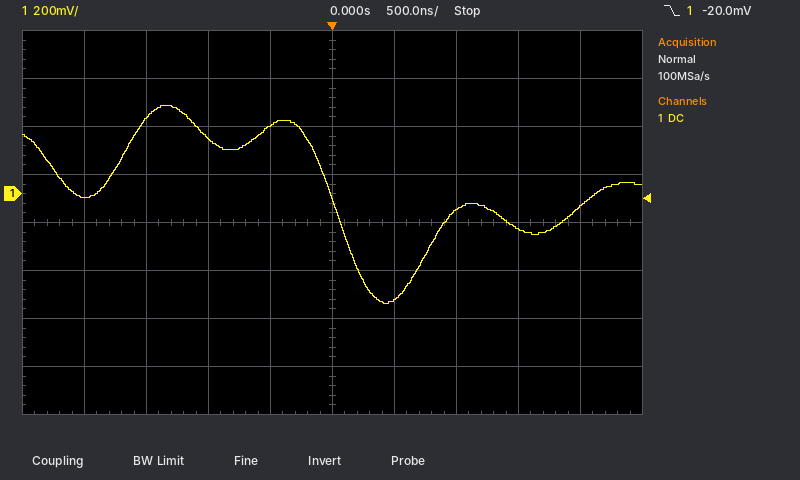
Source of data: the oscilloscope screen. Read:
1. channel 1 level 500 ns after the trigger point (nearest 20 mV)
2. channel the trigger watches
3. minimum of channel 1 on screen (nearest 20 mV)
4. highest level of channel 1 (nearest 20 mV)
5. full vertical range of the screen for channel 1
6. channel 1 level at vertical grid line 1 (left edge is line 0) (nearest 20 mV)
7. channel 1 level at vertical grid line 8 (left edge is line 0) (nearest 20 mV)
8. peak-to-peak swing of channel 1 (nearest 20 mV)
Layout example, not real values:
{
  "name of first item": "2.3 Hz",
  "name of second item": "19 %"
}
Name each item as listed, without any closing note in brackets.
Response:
{
  "channel 1 level 500 ns after the trigger point": "-440 mV",
  "channel the trigger watches": "channel 1",
  "minimum of channel 1 on screen": "-460 mV",
  "highest level of channel 1": "360 mV",
  "full vertical range of the screen for channel 1": "1.6 V",
  "channel 1 level at vertical grid line 1 (left edge is line 0)": "-20 mV",
  "channel 1 level at vertical grid line 8 (left edge is line 0)": "-140 mV",
  "peak-to-peak swing of channel 1": "820 mV"
}
